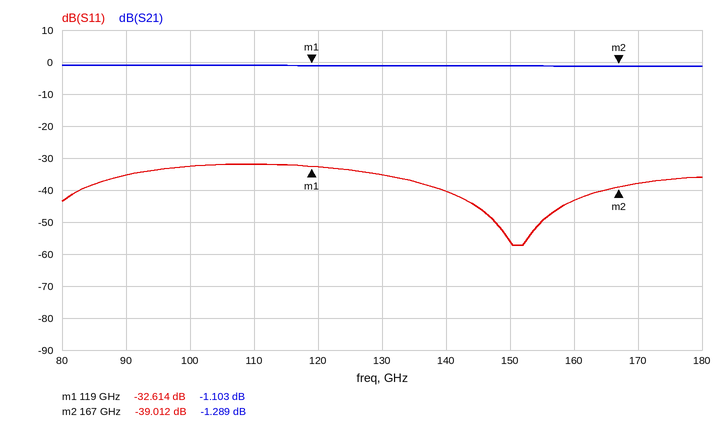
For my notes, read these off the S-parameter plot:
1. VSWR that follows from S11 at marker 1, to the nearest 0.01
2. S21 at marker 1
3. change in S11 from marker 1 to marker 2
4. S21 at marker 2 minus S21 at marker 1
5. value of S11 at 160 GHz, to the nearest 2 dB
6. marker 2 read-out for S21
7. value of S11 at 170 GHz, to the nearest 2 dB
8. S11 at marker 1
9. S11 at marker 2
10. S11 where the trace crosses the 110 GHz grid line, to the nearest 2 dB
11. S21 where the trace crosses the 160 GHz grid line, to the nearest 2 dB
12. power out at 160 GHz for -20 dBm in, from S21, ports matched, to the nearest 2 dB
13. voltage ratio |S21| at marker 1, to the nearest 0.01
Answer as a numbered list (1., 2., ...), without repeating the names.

1. 1.05
2. -1.103 dB
3. -6.398 dB
4. -0.186 dB
5. -44 dB
6. -1.289 dB
7. -38 dB
8. -32.614 dB
9. -39.012 dB
10. -32 dB
11. -2 dB
12. -22 dBm
13. 0.88
